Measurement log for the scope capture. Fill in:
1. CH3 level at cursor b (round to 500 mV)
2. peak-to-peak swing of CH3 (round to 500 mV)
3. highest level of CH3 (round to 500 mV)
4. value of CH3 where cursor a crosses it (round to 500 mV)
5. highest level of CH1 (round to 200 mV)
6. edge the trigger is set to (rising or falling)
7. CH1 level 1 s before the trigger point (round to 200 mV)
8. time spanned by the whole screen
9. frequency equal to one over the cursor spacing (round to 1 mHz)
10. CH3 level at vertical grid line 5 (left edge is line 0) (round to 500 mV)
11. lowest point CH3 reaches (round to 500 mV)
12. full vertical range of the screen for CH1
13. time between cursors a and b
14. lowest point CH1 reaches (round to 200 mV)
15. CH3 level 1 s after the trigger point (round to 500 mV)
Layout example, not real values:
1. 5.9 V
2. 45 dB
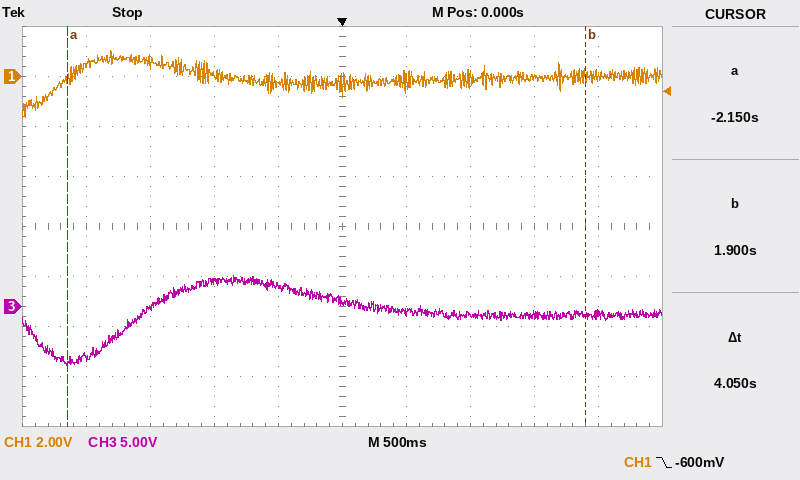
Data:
1. -1.0 V
2. 9.0 V
3. 3.0 V
4. -5.5 V
5. 1.0 V
6. falling
7. 0.0 V
8. 5 s
9. 247 mHz
10. 500 mV
11. -6.0 V
12. 16 V
13. 4.05 s
14. -1.6 V
15. -1.0 V
